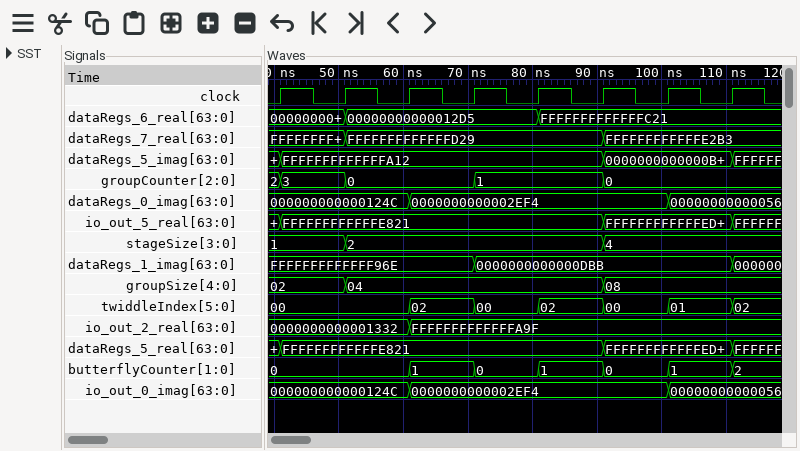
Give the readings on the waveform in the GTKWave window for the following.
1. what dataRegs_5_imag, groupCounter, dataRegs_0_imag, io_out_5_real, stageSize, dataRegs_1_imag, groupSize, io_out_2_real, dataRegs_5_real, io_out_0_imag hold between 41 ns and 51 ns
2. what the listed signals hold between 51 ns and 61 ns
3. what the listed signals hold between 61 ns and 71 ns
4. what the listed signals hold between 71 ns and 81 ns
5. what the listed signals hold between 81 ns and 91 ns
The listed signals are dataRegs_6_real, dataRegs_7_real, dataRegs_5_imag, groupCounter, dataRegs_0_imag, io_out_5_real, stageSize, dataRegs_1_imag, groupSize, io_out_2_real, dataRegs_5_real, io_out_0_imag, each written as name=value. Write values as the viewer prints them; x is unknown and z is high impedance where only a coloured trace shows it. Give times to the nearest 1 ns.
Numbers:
dataRegs_5_imag=FFFFFFFFFFFFFA12, groupCounter=3, dataRegs_0_imag=000000000000124C, io_out_5_real=FFFFFFFFFFFFE821, stageSize=1, dataRegs_1_imag=FFFFFFFFFFFFF96E, groupSize=02, io_out_2_real=0000000000001332, dataRegs_5_real=FFFFFFFFFFFFE821, io_out_0_imag=000000000000124C
dataRegs_6_real=00000000000012D5, dataRegs_7_real=FFFFFFFFFFFFFD29, dataRegs_5_imag=FFFFFFFFFFFFFA12, groupCounter=0, dataRegs_0_imag=000000000000124C, io_out_5_real=FFFFFFFFFFFFE821, stageSize=2, dataRegs_1_imag=FFFFFFFFFFFFF96E, groupSize=04, io_out_2_real=0000000000001332, dataRegs_5_real=FFFFFFFFFFFFE821, io_out_0_imag=000000000000124C
dataRegs_6_real=00000000000012D5, dataRegs_7_real=FFFFFFFFFFFFFD29, dataRegs_5_imag=FFFFFFFFFFFFFA12, groupCounter=0, dataRegs_0_imag=0000000000002EF4, io_out_5_real=FFFFFFFFFFFFE821, stageSize=2, dataRegs_1_imag=FFFFFFFFFFFFF96E, groupSize=04, io_out_2_real=FFFFFFFFFFFFFA9F, dataRegs_5_real=FFFFFFFFFFFFE821, io_out_0_imag=0000000000002EF4
dataRegs_6_real=00000000000012D5, dataRegs_7_real=FFFFFFFFFFFFFD29, dataRegs_5_imag=FFFFFFFFFFFFFA12, groupCounter=1, dataRegs_0_imag=0000000000002EF4, io_out_5_real=FFFFFFFFFFFFE821, stageSize=2, dataRegs_1_imag=0000000000000DBB, groupSize=04, io_out_2_real=FFFFFFFFFFFFFA9F, dataRegs_5_real=FFFFFFFFFFFFE821, io_out_0_imag=0000000000002EF4
dataRegs_6_real=FFFFFFFFFFFFFC21, dataRegs_7_real=FFFFFFFFFFFFFD29, dataRegs_5_imag=FFFFFFFFFFFFFA12, groupCounter=1, dataRegs_0_imag=0000000000002EF4, io_out_5_real=FFFFFFFFFFFFE821, stageSize=2, dataRegs_1_imag=0000000000000DBB, groupSize=04, io_out_2_real=FFFFFFFFFFFFFA9F, dataRegs_5_real=FFFFFFFFFFFFE821, io_out_0_imag=0000000000002EF4
